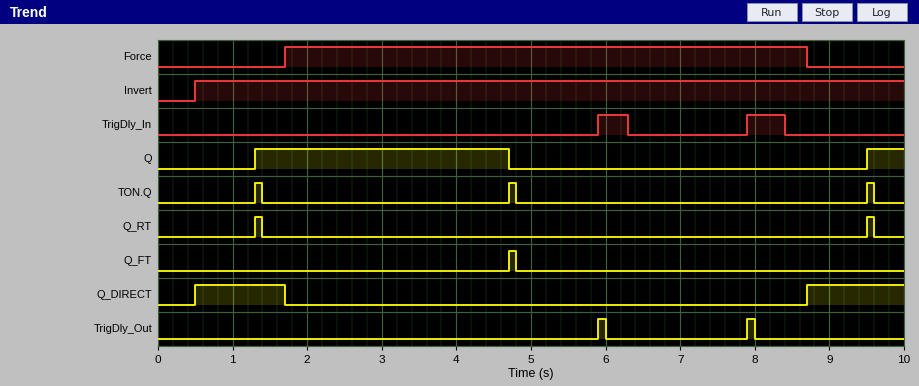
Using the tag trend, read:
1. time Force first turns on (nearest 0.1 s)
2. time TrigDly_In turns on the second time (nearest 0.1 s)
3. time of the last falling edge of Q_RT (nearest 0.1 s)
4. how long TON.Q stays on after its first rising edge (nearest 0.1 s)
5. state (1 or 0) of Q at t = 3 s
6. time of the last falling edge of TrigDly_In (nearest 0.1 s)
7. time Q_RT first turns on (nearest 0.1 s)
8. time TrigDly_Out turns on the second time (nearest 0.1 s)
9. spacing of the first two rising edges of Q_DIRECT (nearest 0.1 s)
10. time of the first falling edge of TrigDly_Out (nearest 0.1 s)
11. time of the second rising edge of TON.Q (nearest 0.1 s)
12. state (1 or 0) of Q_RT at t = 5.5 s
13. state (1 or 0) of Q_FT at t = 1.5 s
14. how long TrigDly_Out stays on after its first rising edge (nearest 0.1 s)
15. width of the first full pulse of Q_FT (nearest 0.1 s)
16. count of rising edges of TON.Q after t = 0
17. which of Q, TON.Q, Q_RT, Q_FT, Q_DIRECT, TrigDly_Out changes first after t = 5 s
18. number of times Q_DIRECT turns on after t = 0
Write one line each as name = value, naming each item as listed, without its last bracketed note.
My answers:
time Force first turns on = 1.7 s
time TrigDly_In turns on the second time = 7.9 s
time of the last falling edge of Q_RT = 9.6 s
how long TON.Q stays on after its first rising edge = 0.1 s
state (1 or 0) of Q at t = 3 s = 1
time of the last falling edge of TrigDly_In = 8.4 s
time Q_RT first turns on = 1.3 s
time TrigDly_Out turns on the second time = 7.9 s
spacing of the first two rising edges of Q_DIRECT = 8.2 s
time of the first falling edge of TrigDly_Out = 6.0 s
time of the second rising edge of TON.Q = 4.7 s
state (1 or 0) of Q_RT at t = 5.5 s = 0
state (1 or 0) of Q_FT at t = 1.5 s = 0
how long TrigDly_Out stays on after its first rising edge = 0.1 s
width of the first full pulse of Q_FT = 0.1 s
count of rising edges of TON.Q after t = 0 = 3
which of Q, TON.Q, Q_RT, Q_FT, Q_DIRECT, TrigDly_Out changes first after t = 5 s = TrigDly_Out
number of times Q_DIRECT turns on after t = 0 = 2
